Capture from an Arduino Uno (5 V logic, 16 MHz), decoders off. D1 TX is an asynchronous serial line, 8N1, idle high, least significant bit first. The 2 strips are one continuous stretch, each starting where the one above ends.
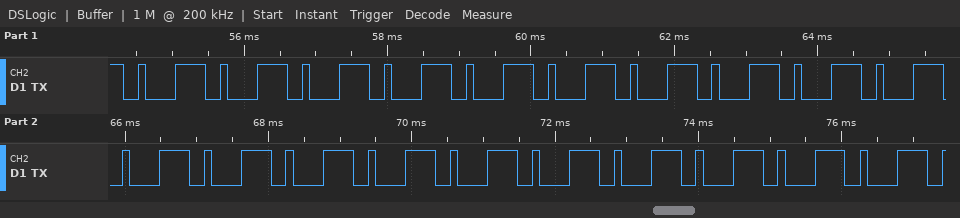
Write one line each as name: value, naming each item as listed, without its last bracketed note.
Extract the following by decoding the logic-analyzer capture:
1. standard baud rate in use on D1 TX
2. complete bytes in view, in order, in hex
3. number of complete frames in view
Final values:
standard baud rate in use on D1 TX: 9600 baud
complete bytes in view, in order, in hex: C2 C2 C2 C2 C2 C2 C2 C2 C2 C2 C2 C2 C2 C2 C2 C2 C2 C2 C2 C2
number of complete frames in view: 20
